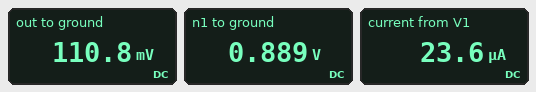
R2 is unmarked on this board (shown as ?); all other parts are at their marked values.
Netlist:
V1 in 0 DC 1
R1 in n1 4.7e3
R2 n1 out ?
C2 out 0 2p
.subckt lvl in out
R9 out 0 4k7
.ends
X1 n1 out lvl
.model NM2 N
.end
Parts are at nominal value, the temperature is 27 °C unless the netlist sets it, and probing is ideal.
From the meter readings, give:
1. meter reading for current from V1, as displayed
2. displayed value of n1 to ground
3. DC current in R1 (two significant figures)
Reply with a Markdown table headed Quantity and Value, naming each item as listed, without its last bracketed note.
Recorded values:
| Quantity | Value |
|---|---|
| meter reading for current from V1, as displayed | 23.6 µA |
| displayed value of n1 to ground | 0.889 V |
| DC current in R1 | 24 µA |
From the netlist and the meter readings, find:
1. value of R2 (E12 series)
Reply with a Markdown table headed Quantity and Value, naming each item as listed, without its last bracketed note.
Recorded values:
| Quantity | Value |
|---|---|
| value of R2 | 33 kΩ |
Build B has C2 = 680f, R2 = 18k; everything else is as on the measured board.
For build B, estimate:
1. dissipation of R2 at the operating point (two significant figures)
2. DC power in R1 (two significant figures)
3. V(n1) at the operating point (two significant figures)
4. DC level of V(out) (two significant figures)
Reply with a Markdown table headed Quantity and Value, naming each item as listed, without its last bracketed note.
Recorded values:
| Quantity | Value |
|---|---|
| dissipation of R2 at the operating point | 24 µW |
| DC power in R1 | 6.3 µW |
| V(n1) at the operating point | 830 mV |
| DC level of V(out) | 170 mV |
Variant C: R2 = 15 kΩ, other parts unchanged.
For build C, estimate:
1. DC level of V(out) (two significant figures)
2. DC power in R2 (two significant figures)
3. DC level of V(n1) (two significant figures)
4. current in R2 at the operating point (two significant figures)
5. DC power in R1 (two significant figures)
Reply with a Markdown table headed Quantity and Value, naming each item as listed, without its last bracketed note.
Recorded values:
| Quantity | Value |
|---|---|
| DC level of V(out) | 190 mV |
| DC power in R2 | 25 µW |
| DC level of V(n1) | 810 mV |
| current in R2 at the operating point | 41 µA |
| DC power in R1 | 7.9 µW |
